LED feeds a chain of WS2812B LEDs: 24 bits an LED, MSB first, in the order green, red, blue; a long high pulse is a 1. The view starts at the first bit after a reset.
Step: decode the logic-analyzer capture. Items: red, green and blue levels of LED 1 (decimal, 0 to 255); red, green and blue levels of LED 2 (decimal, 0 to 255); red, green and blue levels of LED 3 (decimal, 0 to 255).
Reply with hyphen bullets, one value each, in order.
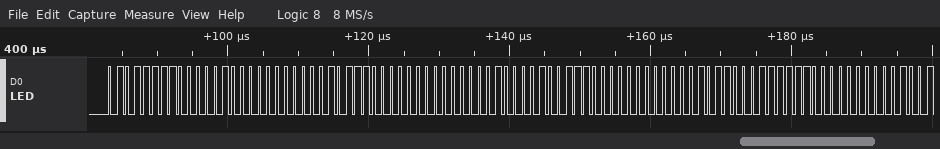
- 4, 95, 0
- 0, 92, 8
- 0, 78, 22
